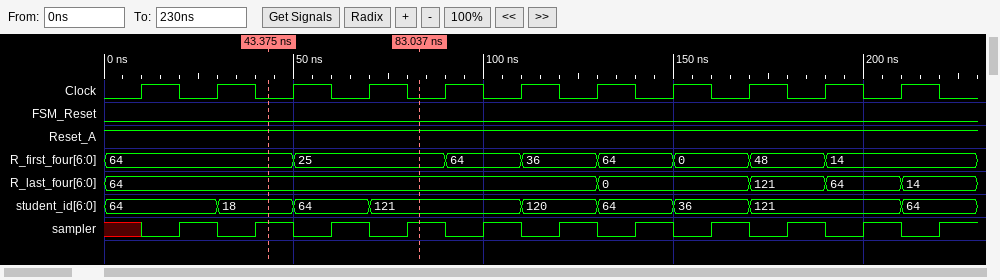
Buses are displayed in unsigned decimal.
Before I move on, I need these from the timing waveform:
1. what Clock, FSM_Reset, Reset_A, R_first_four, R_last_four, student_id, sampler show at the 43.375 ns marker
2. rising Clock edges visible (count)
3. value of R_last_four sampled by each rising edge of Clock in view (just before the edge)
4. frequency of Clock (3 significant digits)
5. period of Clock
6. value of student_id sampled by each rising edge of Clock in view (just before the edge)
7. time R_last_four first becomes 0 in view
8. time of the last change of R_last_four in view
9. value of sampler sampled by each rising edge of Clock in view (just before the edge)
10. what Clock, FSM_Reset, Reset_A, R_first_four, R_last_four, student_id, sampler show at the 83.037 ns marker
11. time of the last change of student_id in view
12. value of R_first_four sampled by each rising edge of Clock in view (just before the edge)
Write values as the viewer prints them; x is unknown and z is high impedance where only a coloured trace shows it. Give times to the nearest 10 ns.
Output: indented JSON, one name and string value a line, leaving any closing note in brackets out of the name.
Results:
{
  "what Clock, FSM_Reset, Reset_A, R_first_four, R_last_four, student_id, sampler show at the 43.375 ns marker": "Clock=0, FSM_Reset=0, Reset_A=1, R_first_four=64, R_last_four=64, student_id=18, sampler=1",
  "rising Clock edges visible": "11",
  "value of R_last_four sampled by each rising edge of Clock in view": "64, 64, 64, 64, 64, 64, 64, 0, 0, 121, 64",
  "frequency of Clock": "50.0 MHz",
  "period of Clock": "20 ns",
  "value of student_id sampled by each rising edge of Clock in view": "64, 64, 18, 64, 121, 121, 120, 64, 36, 121, 121",
  "time R_last_four first becomes 0 in view": "130 ns",
  "time of the last change of R_last_four in view": "210 ns",
  "value of sampler sampled by each rising edge of Clock in view": "x 1 1 1 1 1 1 1 1 1 1",
  "what Clock, FSM_Reset, Reset_A, R_first_four, R_last_four, student_id, sampler show at the 83.037 ns marker": "Clock=0, FSM_Reset=0, Reset_A=1, R_first_four=25, R_last_four=64, student_id=121, sampler=1",
  "time of the last change of student_id in view": "210 ns",
  "value of R_first_four sampled by each rising edge of Clock in view": "64, 64, 64, 25, 25, 64, 36, 64, 0, 48, 14"
}
